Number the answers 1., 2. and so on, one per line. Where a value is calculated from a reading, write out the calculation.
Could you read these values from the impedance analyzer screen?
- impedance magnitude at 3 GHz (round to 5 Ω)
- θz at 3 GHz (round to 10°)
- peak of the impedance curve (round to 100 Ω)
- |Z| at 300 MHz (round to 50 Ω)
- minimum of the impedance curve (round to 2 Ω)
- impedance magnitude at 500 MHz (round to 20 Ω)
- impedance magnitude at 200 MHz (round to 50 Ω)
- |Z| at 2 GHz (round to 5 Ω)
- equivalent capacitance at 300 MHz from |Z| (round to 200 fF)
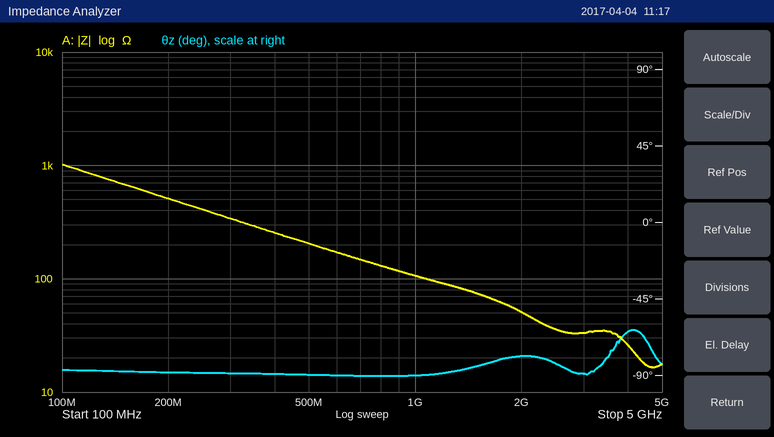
1. 35 Ω
2. -90°
3. 1.0 kΩ
4. 350 Ω
5. 16 Ω
6. 200 Ω
7. 500 Ω
8. 50 Ω
9. C = 1/(2π × 300 MHz × 350 Ω) ≈ 1.52 pF, so 1.6 pF to the nearest 200 fF
